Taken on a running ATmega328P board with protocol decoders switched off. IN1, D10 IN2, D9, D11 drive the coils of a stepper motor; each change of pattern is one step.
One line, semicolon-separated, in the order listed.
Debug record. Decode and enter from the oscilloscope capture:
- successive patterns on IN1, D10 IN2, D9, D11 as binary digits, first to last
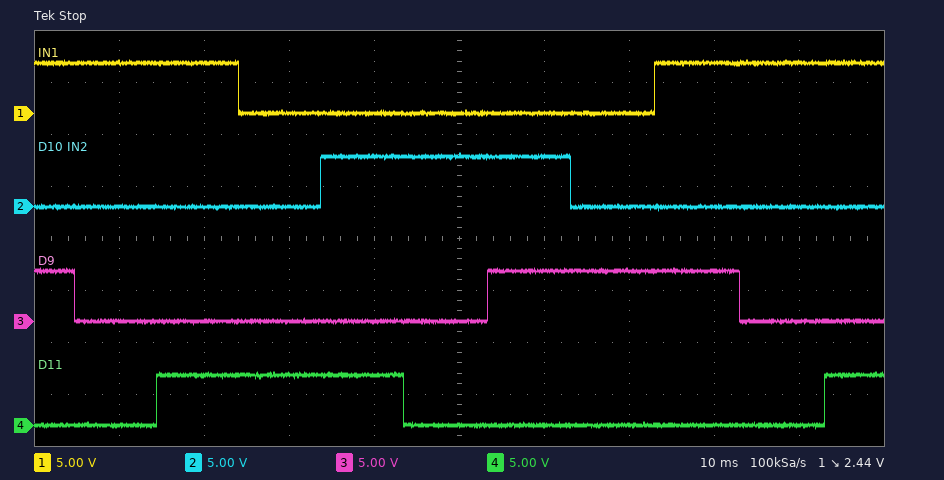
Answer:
1010 1000 1001 0001 0101 0100 0110 0010 1010 1000 1001
